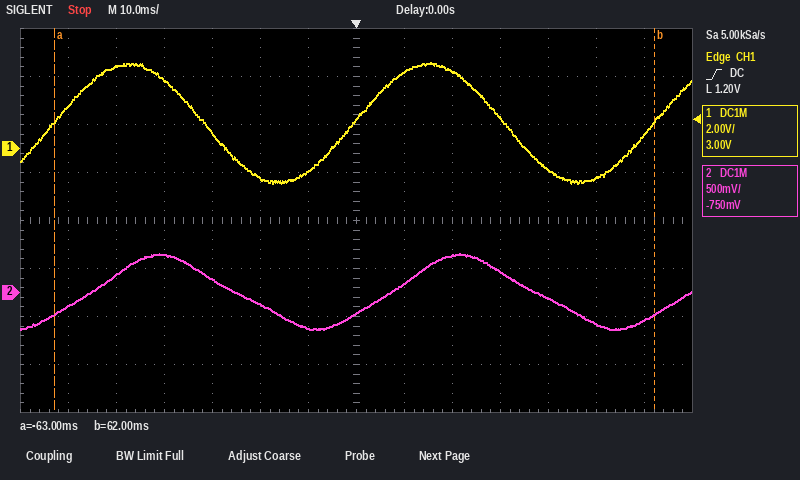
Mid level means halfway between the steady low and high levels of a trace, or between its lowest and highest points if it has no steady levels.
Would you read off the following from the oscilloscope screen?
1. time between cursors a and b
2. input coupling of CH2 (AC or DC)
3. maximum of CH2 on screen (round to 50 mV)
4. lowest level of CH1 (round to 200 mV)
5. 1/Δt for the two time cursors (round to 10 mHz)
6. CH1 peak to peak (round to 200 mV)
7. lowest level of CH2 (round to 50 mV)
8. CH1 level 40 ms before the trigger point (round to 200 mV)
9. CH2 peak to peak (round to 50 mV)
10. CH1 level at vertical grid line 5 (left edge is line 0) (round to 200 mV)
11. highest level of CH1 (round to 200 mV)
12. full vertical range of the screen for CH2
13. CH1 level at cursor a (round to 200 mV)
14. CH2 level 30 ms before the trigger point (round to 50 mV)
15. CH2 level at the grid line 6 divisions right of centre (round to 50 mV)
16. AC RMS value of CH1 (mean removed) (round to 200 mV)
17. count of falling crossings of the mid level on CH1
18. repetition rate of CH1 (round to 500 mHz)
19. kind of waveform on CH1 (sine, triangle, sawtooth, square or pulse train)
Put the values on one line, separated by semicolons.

125 ms; DC; 400 mV; -1.4 V; 8.00 Hz; 5.0 V; -400 mV; 2.8 V; 800 mV; -1.2 V; 3.6 V; 4 V; 1.2 V; 150 mV; -300 mV; 1.8 V; 2; 16.0 Hz; sine
